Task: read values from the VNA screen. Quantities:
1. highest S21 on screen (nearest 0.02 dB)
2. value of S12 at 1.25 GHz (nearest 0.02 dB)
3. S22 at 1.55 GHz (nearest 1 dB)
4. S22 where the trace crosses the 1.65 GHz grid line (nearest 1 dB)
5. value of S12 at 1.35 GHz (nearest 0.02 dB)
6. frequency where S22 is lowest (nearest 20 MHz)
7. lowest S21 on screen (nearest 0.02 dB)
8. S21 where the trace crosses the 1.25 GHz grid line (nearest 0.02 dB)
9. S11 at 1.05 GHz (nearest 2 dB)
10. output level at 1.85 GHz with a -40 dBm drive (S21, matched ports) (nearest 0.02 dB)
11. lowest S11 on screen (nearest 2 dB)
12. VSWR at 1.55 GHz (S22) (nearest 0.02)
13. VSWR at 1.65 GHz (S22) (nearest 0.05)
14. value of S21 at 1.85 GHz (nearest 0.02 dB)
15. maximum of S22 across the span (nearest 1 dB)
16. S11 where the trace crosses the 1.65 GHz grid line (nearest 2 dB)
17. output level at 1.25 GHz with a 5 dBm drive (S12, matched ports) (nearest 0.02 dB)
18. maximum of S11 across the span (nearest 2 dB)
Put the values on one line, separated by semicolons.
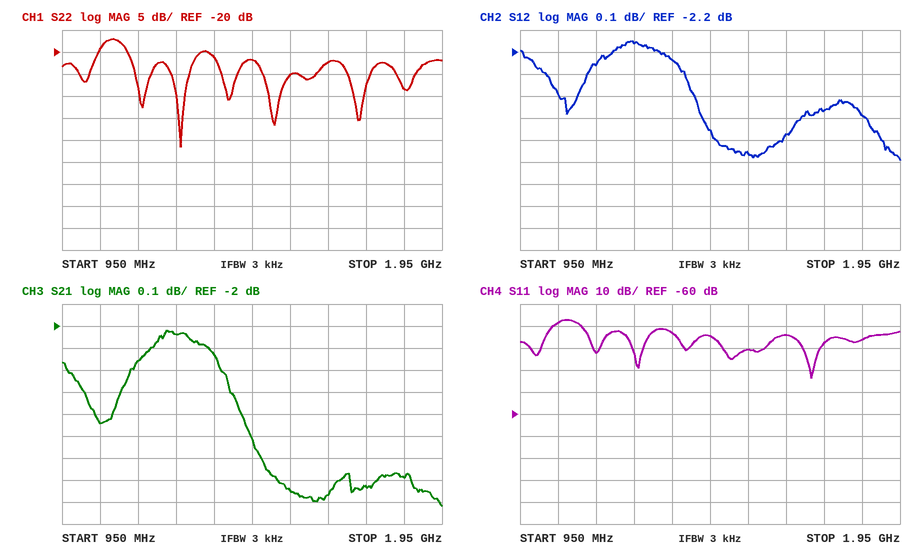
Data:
-2.02 dB; -2.16 dB; -25 dB; -22 dB; -2.24 dB; 1.26 GHz; -2.82 dB; -2.04 dB; -18 dB; -42.68 dBm; -44 dB; 1.12; 1.15; -2.68 dB; -17 dB; -24 dB; 2.84 dBm; -18 dB
